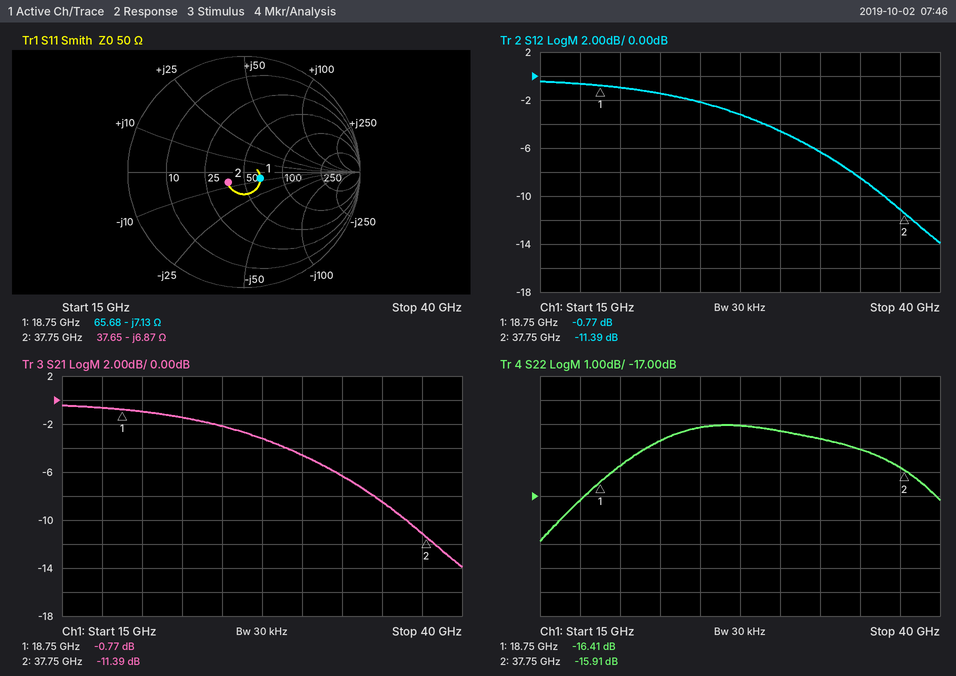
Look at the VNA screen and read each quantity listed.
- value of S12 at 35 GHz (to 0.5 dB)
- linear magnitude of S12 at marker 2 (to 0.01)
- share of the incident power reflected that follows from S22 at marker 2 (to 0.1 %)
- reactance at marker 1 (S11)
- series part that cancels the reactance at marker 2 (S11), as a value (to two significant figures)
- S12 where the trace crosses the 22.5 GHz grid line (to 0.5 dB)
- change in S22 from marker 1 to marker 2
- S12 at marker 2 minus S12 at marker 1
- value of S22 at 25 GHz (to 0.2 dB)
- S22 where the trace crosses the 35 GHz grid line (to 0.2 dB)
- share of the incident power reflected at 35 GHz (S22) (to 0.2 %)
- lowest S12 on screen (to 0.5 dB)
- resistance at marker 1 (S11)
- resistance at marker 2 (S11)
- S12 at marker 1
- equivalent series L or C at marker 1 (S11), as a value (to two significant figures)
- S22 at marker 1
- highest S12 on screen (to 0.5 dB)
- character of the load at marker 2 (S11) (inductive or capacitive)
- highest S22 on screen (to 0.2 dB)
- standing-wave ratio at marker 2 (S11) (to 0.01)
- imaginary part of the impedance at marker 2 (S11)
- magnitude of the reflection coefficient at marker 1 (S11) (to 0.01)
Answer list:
-8.5 dB
0.27
2.6 %
-7.13 Ω
29 pH
-1.5 dB
0.50 dB
-10.62 dB
-14.2 dB
-15.0 dB
3.2 %
-14.0 dB
65.68 Ω
37.65 Ω
-0.77 dB
1.2 pF
-16.41 dB
-0.5 dB
capacitive
-14.0 dB
1.38
-6.87 Ω
0.15
